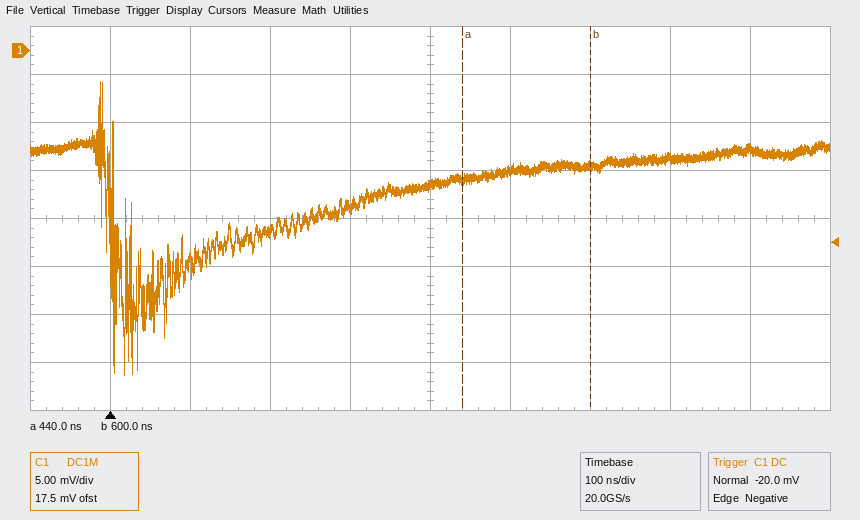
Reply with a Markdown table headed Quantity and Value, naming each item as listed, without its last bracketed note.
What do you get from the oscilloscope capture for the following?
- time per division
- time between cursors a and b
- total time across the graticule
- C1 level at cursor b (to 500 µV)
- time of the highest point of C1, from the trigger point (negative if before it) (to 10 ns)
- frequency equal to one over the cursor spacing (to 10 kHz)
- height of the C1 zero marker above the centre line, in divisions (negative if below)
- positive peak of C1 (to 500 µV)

| Quantity | Value |
|---|---|
| time per division | 100 ns |
| time between cursors a and b | 160 ns |
| total time across the graticule | 1 µs |
| C1 level at cursor b | -12.0 mV |
| time of the highest point of C1, from the trigger point (negative if before it) | -10 ns |
| frequency equal to one over the cursor spacing | 6.25 MHz |
| height of the C1 zero marker above the centre line, in divisions | +3.5 div |
| positive peak of C1 | -3.0 mV |
